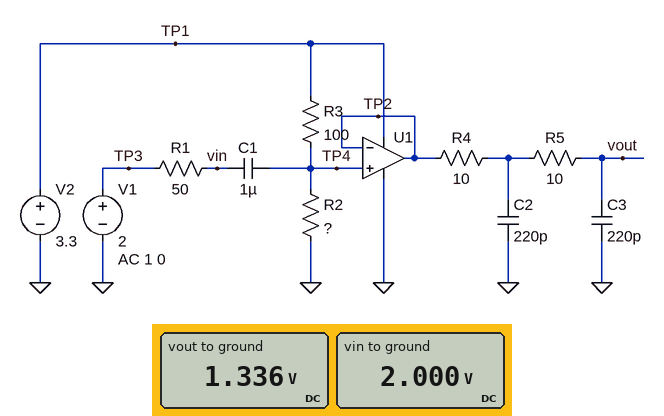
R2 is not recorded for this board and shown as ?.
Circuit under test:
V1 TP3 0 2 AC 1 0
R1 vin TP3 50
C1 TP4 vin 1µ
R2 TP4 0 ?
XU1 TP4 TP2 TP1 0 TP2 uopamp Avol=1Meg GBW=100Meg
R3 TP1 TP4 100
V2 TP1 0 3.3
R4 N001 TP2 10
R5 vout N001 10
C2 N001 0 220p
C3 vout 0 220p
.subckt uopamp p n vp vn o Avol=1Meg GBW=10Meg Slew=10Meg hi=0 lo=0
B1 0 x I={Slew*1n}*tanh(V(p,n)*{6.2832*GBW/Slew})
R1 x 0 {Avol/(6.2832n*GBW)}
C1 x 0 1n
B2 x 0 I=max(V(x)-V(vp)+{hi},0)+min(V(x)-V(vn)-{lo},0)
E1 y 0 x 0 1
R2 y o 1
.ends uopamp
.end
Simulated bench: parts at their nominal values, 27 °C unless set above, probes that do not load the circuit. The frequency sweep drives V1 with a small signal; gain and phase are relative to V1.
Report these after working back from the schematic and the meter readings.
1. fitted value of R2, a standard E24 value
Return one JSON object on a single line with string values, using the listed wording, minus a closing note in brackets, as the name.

{"fitted value of R2, a standard E24 value": "68 Ω"}
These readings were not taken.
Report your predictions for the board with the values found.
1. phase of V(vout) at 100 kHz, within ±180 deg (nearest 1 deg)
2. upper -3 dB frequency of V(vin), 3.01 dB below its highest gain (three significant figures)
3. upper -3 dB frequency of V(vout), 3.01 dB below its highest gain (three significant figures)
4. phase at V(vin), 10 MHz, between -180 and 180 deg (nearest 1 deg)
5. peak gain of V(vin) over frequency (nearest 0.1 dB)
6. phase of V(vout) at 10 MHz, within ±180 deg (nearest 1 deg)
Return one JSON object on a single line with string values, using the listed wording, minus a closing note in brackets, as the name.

{"phase of V(vout) at 100 kHz, within ±180 deg": "1 deg", "upper -3 dB frequency of V(vin), 3.01 dB below its highest gain": "2.27 kHz", "upper -3 dB frequency of V(vout), 3.01 dB below its highest gain": "25.8 MHz", "phase at V(vin), 10 MHz, between -180 and 180 deg": "0 deg", "peak gain of V(vin) over frequency": "0 dB", "phase of V(vout) at 10 MHz, within ±180 deg": "-29 deg"}
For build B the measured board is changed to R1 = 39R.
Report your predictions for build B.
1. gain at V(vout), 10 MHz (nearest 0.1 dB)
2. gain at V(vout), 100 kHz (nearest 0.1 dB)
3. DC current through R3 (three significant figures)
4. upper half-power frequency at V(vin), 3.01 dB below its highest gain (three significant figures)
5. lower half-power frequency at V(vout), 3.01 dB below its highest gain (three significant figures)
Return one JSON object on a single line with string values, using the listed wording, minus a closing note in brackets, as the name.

{"gain at V(vout), 10 MHz": "-6.4 dB", "gain at V(vout), 100 kHz": "-5.9 dB", "DC current through R3": "19.6 mA", "upper half-power frequency at V(vin), 3.01 dB below its highest gain": "2.89 kHz", "lower half-power frequency at V(vout), 3.01 dB below its highest gain": "2.00 kHz"}
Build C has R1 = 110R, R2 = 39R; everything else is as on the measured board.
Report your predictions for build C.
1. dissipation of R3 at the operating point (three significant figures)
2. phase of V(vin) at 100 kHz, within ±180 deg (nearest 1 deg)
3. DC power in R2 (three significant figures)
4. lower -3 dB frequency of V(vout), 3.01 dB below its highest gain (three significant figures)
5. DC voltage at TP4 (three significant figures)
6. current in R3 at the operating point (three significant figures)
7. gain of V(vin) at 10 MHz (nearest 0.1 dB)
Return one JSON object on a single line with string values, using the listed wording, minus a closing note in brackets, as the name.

{"dissipation of R3 at the operating point": "56.4 mW", "phase of V(vin) at 100 kHz, within ±180 deg": "-3 deg", "DC power in R2": "22.0 mW", "lower -3 dB frequency of V(vout), 3.01 dB below its highest gain": "1.15 kHz", "DC voltage at TP4": "926 mV", "current in R3 at the operating point": "23.7 mA", "gain of V(vin) at 10 MHz": "-13.8 dB"}
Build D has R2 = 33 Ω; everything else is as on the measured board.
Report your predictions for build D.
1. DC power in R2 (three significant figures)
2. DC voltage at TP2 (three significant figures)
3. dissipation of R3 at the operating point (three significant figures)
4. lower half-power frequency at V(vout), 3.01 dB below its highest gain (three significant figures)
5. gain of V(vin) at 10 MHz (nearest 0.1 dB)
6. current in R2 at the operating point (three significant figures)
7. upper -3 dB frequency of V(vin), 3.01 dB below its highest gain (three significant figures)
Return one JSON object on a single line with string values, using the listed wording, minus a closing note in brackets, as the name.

{"DC power in R2": "20.3 mW", "DC voltage at TP2": "819 mV", "dissipation of R3 at the operating point": "61.6 mW", "lower half-power frequency at V(vout), 3.01 dB below its highest gain": "2.13 kHz", "gain of V(vin) at 10 MHz": "-9.6 dB", "current in R2 at the operating point": "24.8 mA", "upper -3 dB frequency of V(vin), 3.01 dB below its highest gain": "2.41 kHz"}
